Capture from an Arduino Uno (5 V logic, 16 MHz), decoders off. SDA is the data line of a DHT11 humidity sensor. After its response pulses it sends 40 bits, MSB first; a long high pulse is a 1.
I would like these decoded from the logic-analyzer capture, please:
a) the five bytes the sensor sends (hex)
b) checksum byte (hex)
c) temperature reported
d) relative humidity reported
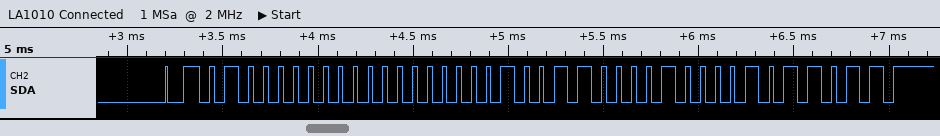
40 00 13 08 5B
0x5B
19.8 °C
64 %
